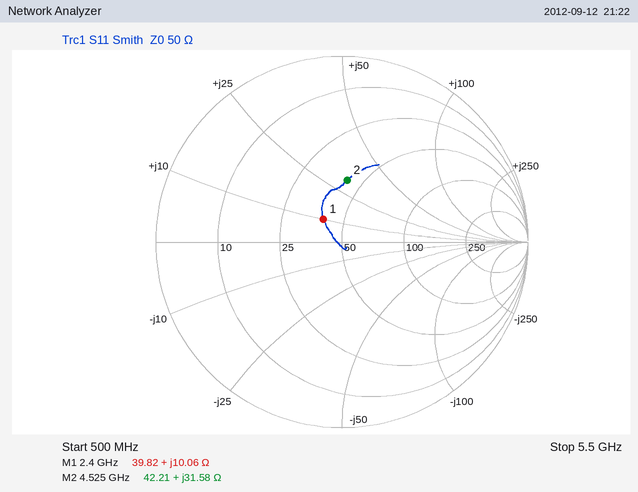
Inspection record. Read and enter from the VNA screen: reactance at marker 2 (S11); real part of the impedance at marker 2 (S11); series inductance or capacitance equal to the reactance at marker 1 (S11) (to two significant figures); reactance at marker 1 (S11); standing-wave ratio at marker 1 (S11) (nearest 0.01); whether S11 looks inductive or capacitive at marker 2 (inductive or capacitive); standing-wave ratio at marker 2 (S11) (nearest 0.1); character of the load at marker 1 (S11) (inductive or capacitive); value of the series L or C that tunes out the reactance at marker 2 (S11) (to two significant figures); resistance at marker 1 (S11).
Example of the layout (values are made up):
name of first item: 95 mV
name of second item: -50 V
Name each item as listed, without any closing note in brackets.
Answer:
reactance at marker 2: +31.58 Ω
real part of the impedance at marker 2: 42.21 Ω
series inductance or capacitance equal to the reactance at marker 1 (S11): 670 pH
reactance at marker 1: +10.06 Ω
standing-wave ratio at marker 1 (S11): 1.38
whether S11 looks inductive or capacitive at marker 2: inductive
standing-wave ratio at marker 2 (S11): 2.0
character of the load at marker 1 (S11): inductive
value of the series L or C that tunes out the reactance at marker 2 (S11): 1.1 pF
resistance at marker 1: 39.82 Ω
